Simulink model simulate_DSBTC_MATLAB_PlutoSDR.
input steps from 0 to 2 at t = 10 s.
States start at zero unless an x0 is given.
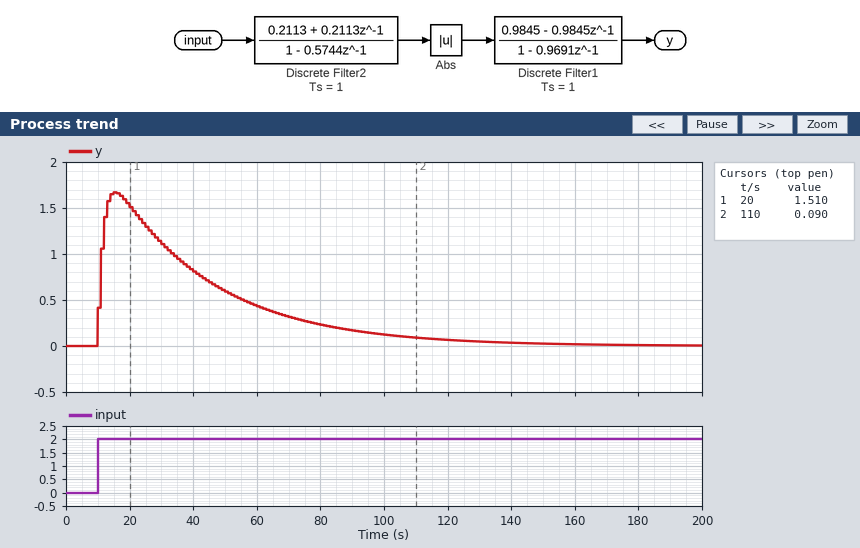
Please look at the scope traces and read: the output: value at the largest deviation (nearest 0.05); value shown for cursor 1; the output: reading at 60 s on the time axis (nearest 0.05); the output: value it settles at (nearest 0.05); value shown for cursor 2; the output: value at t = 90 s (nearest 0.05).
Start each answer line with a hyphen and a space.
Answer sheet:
- 1.65
- 1.510
- 0.45
- 0.00
- 0.090
- 0.15
